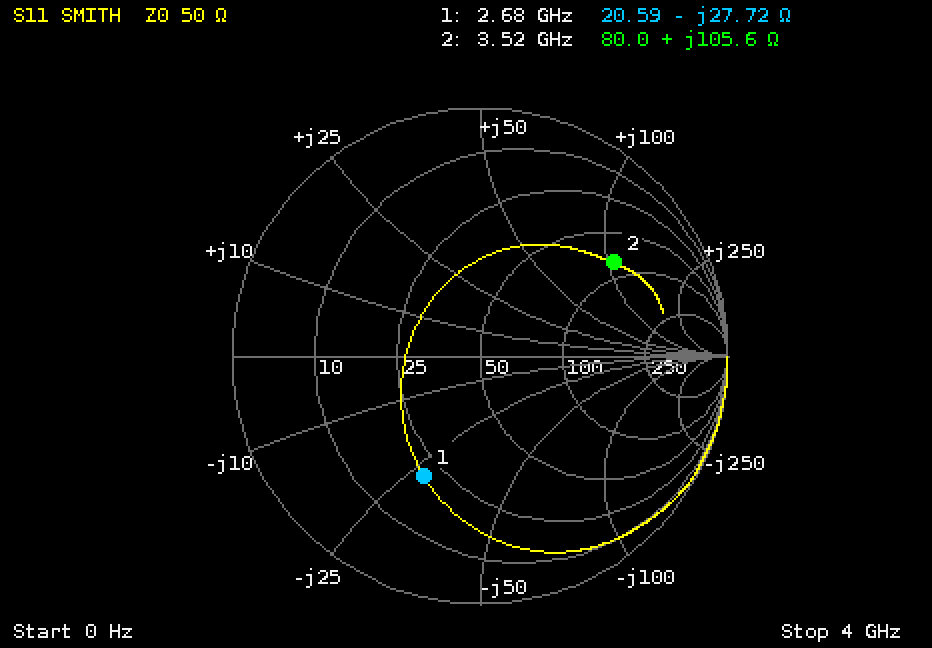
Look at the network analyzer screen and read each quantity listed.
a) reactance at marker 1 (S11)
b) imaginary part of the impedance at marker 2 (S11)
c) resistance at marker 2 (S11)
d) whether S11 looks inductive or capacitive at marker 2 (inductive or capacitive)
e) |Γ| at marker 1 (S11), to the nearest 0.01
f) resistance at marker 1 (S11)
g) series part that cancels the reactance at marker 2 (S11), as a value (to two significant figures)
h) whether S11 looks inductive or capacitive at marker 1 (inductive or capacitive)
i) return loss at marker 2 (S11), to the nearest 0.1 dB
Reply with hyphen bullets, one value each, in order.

- -27.72 Ω
- +105.6 Ω
- 80.0 Ω
- inductive
- 0.53
- 20.59 Ω
- 430 fF
- capacitive
- 3.7 dB
